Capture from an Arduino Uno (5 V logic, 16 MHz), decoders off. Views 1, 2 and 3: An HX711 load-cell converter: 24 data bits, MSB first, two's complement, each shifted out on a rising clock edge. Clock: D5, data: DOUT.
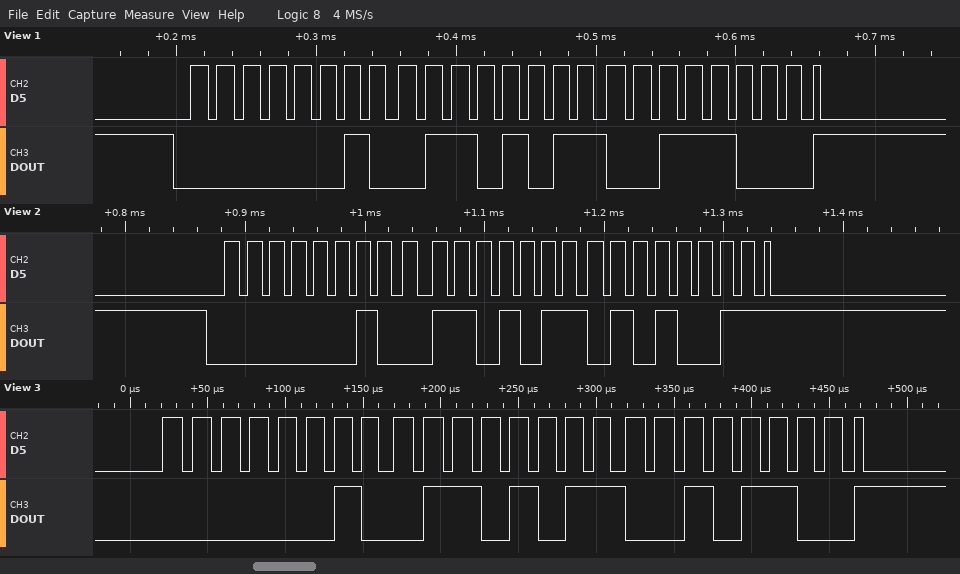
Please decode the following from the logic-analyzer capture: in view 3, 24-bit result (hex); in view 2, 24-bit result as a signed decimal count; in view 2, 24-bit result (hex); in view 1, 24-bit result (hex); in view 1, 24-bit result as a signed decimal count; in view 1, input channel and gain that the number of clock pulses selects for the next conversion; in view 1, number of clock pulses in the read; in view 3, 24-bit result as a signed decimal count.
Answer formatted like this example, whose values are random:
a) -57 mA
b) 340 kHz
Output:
a) 0x026B2C
b) 158547
c) 0x026B53
d) 0x026B38
e) 158520
f) channel A, gain 128
g) 25
h) 158508
